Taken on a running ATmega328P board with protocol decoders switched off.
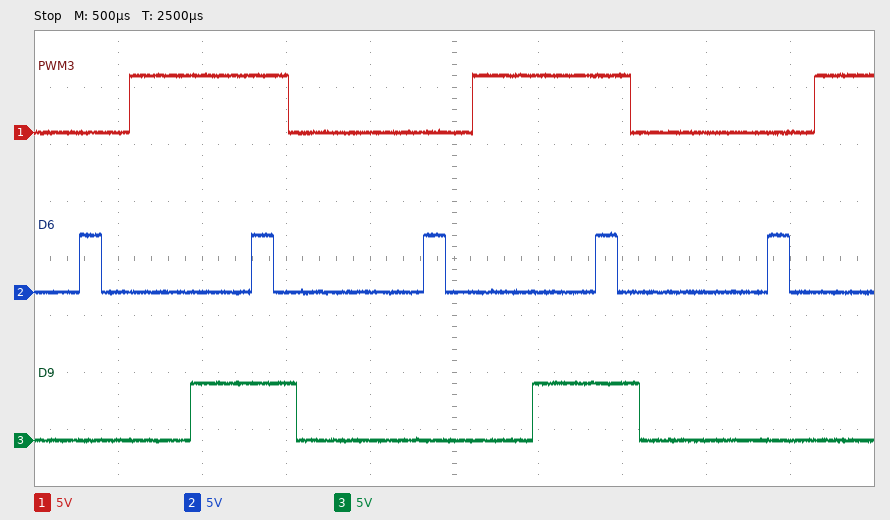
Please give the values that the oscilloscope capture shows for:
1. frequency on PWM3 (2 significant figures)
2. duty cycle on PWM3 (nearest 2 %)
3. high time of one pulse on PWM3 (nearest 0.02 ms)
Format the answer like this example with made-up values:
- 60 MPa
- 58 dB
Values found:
- 490 Hz
- 46 %
- 0.94 ms
